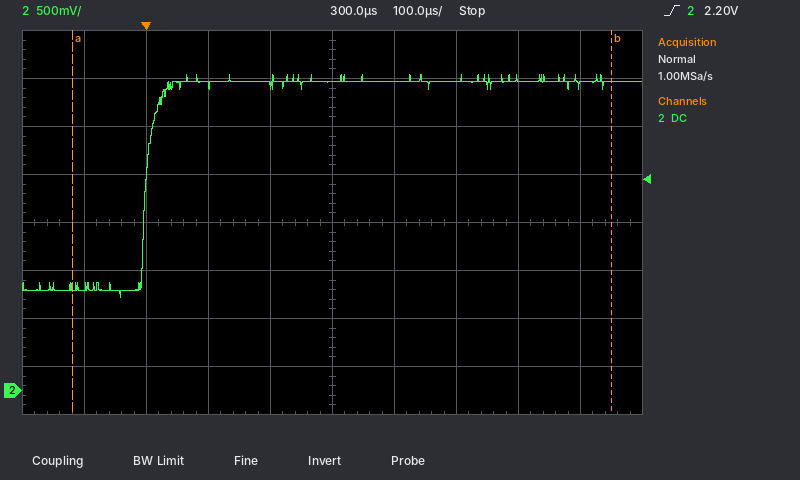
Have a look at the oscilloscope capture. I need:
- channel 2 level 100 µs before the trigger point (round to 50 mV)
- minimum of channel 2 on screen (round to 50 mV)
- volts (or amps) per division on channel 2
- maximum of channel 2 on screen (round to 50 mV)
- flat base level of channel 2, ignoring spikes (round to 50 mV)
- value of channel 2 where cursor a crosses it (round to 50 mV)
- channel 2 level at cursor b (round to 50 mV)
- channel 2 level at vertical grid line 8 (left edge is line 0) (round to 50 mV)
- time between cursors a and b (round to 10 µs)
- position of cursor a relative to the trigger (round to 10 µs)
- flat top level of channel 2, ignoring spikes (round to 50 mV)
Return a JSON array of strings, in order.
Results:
["1.10 V", "950 mV", "500 mV", "3.30 V", "1.05 V", "1.10 V", "3.20 V", "3.25 V", "870 µs", "-120 µs", "3.20 V"]
